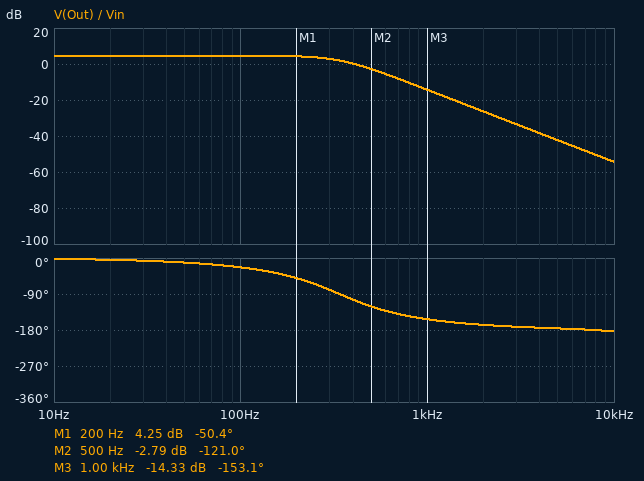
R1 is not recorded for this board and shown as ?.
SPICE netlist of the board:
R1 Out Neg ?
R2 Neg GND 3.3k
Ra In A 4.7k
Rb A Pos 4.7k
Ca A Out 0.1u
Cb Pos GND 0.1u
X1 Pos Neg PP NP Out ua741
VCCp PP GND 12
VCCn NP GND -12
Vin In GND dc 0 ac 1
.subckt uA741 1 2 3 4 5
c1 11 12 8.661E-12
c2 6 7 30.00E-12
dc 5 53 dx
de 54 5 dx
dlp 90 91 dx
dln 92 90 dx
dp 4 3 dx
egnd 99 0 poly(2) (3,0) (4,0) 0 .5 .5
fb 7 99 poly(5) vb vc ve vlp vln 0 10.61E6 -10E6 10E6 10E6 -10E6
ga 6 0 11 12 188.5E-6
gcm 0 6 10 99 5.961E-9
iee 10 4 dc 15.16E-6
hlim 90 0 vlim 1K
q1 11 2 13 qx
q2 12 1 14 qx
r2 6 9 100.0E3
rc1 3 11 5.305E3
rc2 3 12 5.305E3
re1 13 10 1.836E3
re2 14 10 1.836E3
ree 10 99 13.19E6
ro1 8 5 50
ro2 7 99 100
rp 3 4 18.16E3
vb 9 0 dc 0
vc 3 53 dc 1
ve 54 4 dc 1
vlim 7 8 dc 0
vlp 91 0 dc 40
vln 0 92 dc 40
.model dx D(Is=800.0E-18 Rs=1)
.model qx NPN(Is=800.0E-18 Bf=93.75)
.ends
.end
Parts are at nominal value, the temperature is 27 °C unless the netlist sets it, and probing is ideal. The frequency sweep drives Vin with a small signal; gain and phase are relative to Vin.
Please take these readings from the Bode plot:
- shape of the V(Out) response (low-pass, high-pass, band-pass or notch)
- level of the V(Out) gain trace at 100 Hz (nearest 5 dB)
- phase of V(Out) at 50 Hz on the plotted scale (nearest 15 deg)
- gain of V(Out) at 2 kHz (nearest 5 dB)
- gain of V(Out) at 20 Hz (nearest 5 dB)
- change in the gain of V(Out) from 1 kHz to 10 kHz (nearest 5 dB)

low-pass
5 dB
-15 deg
-25 dB
5 dB
-40 dB
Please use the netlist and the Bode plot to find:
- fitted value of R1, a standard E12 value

2.2 kΩ
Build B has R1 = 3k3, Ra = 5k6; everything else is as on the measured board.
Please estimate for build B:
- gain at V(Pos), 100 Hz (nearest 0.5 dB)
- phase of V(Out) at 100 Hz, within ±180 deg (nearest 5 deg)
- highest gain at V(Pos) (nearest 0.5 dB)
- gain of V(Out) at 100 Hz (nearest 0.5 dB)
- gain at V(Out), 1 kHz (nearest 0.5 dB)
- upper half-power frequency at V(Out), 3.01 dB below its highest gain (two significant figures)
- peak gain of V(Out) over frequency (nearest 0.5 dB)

0.5 dB
-20 deg
2.0 dB
6.5 dB
-14.0 dB
370 Hz
8.0 dB
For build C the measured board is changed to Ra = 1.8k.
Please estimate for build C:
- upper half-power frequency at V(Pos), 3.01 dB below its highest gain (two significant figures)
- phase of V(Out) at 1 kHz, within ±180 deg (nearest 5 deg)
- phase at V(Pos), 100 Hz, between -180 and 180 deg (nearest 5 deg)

400 Hz
-125 deg
-20 deg
